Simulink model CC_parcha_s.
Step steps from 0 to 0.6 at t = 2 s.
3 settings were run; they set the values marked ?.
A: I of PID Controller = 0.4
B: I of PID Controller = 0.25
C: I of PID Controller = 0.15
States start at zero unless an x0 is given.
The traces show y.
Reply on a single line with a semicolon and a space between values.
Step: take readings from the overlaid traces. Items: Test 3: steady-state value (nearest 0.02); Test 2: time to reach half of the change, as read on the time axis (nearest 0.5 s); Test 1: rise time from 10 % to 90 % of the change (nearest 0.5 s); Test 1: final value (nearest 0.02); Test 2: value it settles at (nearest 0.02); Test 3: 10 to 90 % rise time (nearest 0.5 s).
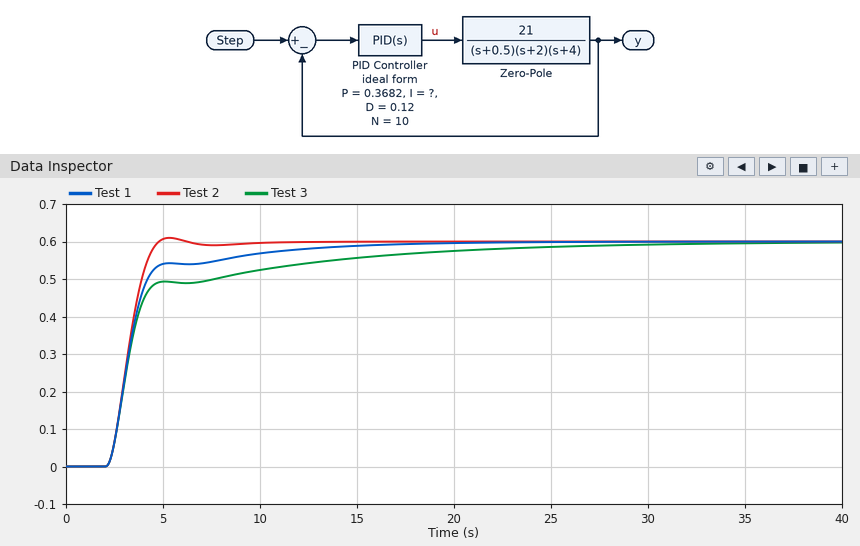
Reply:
0.60; 3.0 s; 2.5 s; 0.60; 0.60; 9.5 s
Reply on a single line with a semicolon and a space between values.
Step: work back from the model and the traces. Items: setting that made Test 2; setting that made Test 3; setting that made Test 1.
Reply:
A; C; B
